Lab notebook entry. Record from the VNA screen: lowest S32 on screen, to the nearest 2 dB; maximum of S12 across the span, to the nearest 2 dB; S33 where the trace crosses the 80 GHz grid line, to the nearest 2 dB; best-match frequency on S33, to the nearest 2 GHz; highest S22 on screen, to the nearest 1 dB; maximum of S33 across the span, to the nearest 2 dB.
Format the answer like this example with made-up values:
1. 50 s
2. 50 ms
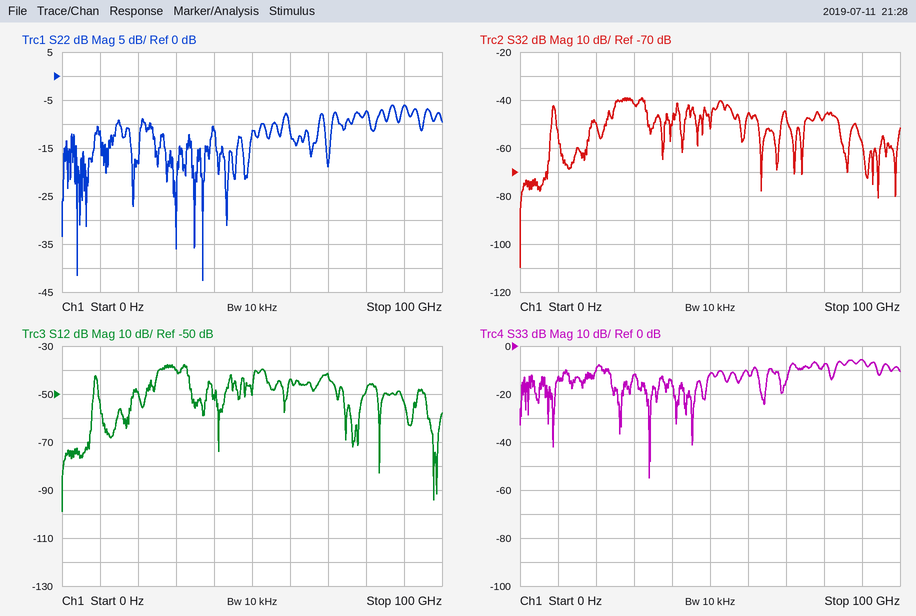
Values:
1. -110 dB
2. -38 dB
3. -8 dB
4. 34 GHz
5. -6 dB
6. -6 dB
